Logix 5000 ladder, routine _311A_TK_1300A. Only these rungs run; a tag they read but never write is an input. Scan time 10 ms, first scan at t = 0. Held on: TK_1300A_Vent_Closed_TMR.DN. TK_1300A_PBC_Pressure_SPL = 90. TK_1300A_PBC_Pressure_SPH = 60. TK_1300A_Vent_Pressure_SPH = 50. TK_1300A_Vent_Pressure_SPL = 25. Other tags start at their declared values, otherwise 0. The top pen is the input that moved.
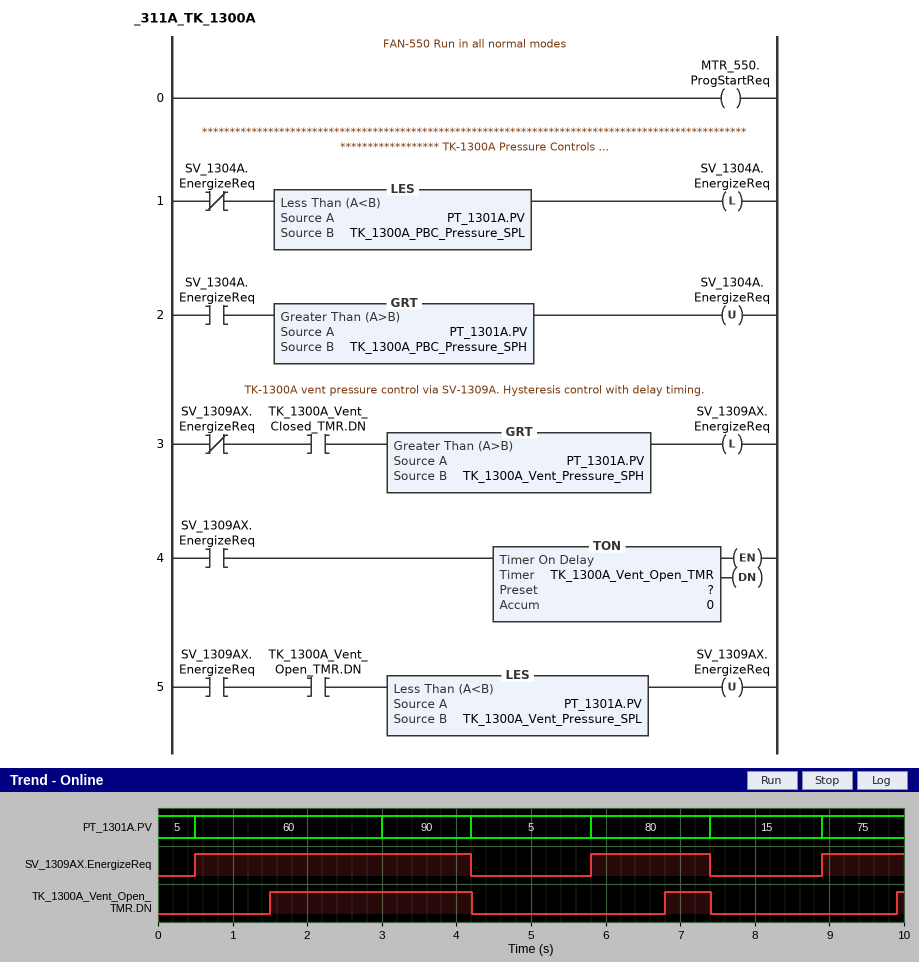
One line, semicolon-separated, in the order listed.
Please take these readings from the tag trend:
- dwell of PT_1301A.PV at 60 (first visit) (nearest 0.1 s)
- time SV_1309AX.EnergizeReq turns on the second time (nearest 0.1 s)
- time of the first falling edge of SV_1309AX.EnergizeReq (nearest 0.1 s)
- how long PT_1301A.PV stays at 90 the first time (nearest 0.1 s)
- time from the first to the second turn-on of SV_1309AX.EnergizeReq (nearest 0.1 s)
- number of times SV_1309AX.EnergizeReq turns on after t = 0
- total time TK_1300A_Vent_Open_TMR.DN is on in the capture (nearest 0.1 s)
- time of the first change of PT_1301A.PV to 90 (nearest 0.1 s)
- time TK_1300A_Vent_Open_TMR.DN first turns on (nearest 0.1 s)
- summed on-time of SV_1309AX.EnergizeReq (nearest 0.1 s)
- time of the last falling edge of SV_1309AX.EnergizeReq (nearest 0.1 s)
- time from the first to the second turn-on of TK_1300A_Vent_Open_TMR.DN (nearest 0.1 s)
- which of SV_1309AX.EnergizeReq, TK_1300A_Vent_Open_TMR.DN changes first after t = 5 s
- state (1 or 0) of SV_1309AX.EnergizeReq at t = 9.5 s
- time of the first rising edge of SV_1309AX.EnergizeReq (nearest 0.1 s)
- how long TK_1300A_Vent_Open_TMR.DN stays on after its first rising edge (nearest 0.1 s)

2.5 s; 5.8 s; 4.2 s; 1.2 s; 5.3 s; 3; 3.4 s; 3.0 s; 1.5 s; 6.4 s; 7.4 s; 5.3 s; SV_1309AX.EnergizeReq; 1; 0.5 s; 2.7 s
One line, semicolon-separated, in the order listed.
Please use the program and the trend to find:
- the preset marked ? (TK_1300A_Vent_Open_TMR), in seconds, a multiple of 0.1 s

1.0 s
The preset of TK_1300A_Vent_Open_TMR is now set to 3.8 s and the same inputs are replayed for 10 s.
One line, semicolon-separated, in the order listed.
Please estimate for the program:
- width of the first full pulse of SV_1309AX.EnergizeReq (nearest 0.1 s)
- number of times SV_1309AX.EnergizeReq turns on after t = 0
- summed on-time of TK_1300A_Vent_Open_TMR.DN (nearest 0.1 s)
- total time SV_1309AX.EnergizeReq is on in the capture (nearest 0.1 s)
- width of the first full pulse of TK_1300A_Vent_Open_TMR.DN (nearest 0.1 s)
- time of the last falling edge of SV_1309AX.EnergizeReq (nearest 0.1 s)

3.8 s; 2; 0.4 s; 8.0 s; 0.0 s; 4.3 s
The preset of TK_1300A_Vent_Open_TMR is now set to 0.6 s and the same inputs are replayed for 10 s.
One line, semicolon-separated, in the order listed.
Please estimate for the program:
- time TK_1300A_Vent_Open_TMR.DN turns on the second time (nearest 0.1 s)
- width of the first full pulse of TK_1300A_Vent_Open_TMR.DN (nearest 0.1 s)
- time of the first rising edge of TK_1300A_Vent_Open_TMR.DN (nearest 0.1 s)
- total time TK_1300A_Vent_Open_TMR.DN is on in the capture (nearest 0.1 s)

6.4 s; 3.1 s; 1.1 s; 4.6 s
